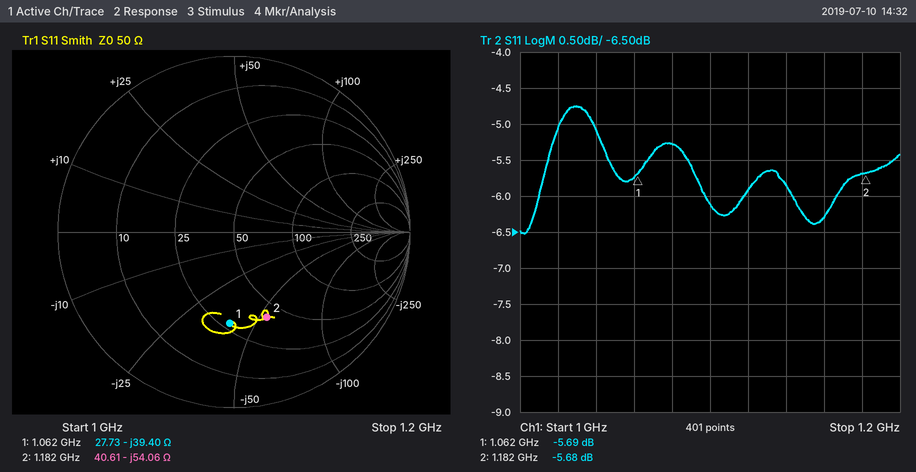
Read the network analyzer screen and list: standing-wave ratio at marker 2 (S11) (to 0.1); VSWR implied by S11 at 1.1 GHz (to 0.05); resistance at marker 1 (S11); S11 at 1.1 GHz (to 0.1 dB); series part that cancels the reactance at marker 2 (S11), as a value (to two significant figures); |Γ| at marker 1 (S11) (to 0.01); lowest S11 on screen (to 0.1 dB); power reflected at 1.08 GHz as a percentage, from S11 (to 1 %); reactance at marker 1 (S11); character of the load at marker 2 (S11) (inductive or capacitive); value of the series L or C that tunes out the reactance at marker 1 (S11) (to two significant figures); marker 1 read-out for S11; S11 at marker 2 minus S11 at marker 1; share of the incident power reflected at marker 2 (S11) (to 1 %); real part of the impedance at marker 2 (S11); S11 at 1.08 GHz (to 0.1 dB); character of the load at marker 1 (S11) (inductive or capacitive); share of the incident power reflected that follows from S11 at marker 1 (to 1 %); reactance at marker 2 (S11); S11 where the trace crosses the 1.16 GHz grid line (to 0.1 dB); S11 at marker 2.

3.2
2.95
27.73 Ω
-6.1 dB
7.3 nH
0.52
-6.5 dB
30 %
-39.40 Ω
capacitive
5.9 nH
-5.69 dB
0.01 dB
27 %
40.61 Ω
-5.3 dB
capacitive
27 %
-54.06 Ω
-6.3 dB
-5.68 dB
